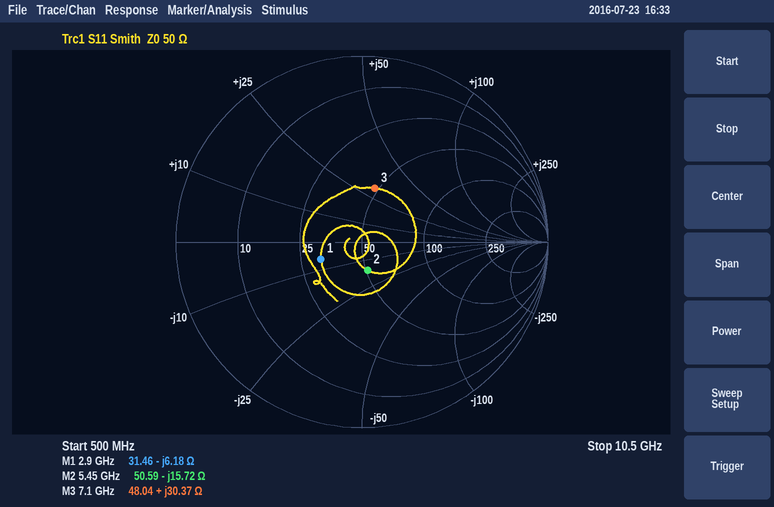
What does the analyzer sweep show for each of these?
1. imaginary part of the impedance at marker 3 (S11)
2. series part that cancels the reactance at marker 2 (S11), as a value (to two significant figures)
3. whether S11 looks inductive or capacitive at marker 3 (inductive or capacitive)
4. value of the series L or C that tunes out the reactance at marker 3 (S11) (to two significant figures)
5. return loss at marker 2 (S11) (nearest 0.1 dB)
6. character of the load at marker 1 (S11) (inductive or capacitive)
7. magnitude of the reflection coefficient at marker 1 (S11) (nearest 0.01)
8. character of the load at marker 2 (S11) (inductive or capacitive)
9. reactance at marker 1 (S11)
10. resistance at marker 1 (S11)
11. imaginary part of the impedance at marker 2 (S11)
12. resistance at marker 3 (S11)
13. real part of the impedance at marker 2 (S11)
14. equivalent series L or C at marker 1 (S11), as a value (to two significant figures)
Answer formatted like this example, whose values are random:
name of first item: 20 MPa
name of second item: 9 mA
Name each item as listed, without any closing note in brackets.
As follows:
imaginary part of the impedance at marker 3: +30.37 Ω
series part that cancels the reactance at marker 2 (S11), as a value: 460 pH
whether S11 looks inductive or capacitive at marker 3: inductive
value of the series L or C that tunes out the reactance at marker 3 (S11): 740 fF
return loss at marker 2 (S11): 16.2 dB
character of the load at marker 1 (S11): capacitive
magnitude of the reflection coefficient at marker 1 (S11): 0.24
character of the load at marker 2 (S11): capacitive
reactance at marker 1: -6.18 Ω
resistance at marker 1: 31.46 Ω
imaginary part of the impedance at marker 2: -15.72 Ω
resistance at marker 3: 48.04 Ω
real part of the impedance at marker 2: 50.59 Ω
equivalent series L or C at marker 1 (S11), as a value: 8.9 pF
